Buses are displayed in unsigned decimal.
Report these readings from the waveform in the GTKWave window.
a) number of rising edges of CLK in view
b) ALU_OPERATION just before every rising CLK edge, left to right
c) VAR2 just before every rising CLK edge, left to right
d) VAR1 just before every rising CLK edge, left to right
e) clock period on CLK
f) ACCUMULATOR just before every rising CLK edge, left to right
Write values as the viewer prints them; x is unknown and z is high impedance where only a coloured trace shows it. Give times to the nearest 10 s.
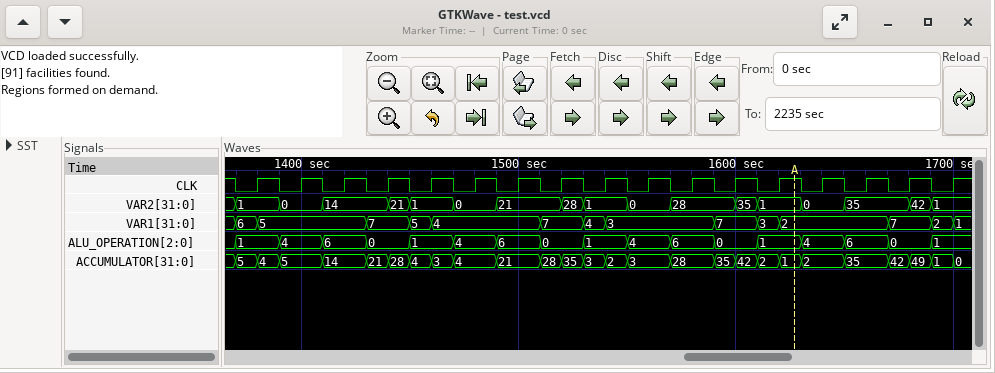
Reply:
17
1, 4, 6, 0, 1, 4, 6, 0, 1, 4, 6, 0, 1, 4, 6, 0, 1
1, 0, 14, 14, 1, 0, 21, 21, 1, 0, 28, 28, 1, 0, 35, 35, 1
6, 5, 5, 7, 5, 4, 4, 7, 4, 3, 3, 7, 3, 2, 2, 7, 2
20 s
5, 5, 14, 21, 4, 4, 21, 28, 3, 3, 28, 35, 2, 2, 35, 42, 1
